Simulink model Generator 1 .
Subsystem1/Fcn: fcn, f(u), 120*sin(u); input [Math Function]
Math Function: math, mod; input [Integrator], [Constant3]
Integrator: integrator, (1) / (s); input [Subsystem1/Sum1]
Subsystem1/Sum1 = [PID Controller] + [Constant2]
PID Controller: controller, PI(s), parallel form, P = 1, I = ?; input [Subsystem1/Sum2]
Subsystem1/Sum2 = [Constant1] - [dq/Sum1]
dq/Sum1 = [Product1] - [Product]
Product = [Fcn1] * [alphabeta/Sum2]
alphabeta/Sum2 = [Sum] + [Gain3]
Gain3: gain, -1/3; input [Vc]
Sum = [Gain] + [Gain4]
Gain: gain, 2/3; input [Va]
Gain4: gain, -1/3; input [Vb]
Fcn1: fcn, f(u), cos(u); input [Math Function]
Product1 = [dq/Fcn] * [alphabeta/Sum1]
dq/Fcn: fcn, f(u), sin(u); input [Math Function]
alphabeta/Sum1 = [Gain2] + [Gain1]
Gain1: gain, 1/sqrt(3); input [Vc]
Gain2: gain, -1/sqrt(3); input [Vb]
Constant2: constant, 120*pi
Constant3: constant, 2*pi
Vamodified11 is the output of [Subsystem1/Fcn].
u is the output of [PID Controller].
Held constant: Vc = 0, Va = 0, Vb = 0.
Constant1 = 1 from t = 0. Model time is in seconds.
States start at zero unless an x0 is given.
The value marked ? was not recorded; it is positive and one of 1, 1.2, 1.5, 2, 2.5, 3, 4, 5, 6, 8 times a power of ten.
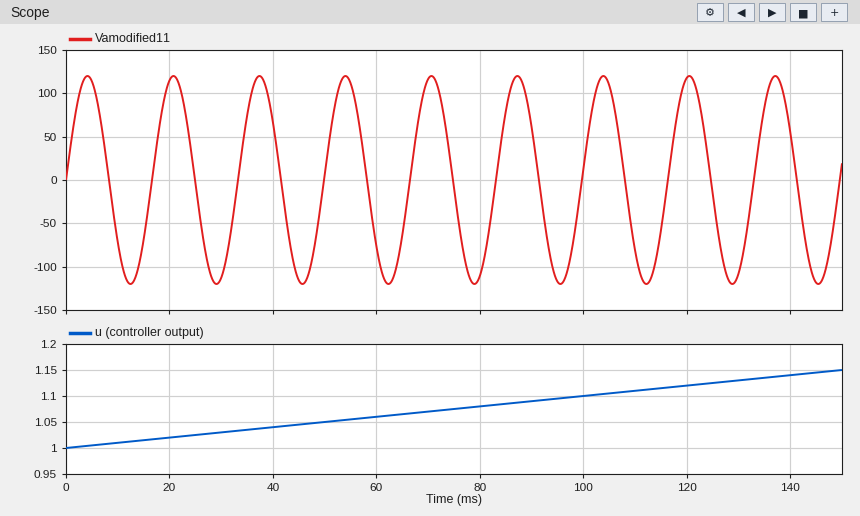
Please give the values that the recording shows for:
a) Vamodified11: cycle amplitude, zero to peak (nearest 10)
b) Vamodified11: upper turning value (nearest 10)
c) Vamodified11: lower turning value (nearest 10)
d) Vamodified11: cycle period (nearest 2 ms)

120
120
-120
16 ms
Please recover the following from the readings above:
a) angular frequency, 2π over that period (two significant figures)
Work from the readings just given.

0.39 rad/ms
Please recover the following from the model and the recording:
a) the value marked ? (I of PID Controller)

1
